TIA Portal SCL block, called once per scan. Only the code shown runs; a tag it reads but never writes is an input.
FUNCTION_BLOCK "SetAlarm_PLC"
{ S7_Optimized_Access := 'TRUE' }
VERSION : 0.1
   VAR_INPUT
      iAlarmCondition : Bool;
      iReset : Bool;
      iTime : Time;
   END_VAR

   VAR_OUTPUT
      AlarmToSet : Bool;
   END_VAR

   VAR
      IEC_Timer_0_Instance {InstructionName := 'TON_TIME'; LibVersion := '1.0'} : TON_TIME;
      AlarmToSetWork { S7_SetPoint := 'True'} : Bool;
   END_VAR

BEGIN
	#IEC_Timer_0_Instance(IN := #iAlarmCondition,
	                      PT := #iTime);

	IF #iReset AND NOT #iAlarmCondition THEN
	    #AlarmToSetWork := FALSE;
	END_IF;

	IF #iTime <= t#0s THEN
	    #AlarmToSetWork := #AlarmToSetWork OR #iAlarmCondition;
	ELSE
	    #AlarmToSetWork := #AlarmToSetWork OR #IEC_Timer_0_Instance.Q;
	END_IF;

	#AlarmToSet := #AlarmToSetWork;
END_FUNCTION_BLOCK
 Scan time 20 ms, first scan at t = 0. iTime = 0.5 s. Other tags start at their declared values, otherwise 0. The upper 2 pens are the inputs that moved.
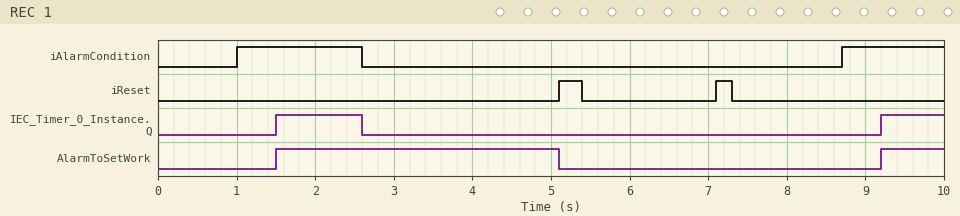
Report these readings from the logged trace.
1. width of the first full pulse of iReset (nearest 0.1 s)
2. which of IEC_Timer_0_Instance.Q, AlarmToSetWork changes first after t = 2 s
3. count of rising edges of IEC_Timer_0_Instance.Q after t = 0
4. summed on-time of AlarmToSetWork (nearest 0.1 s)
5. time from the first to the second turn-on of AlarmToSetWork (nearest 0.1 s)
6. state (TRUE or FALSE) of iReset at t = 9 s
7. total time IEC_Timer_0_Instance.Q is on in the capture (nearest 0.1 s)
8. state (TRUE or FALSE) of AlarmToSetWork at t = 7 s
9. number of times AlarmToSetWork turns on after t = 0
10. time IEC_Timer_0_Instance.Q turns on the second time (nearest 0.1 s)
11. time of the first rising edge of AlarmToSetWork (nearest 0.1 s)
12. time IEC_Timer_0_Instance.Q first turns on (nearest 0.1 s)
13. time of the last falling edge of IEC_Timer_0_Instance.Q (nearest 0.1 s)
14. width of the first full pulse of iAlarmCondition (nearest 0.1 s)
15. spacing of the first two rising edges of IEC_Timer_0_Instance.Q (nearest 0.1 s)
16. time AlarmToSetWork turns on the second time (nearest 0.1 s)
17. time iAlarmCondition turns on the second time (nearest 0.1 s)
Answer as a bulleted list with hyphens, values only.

- 0.3 s
- IEC_Timer_0_Instance.Q
- 2
- 4.4 s
- 7.7 s
- FALSE
- 1.9 s
- FALSE
- 2
- 9.2 s
- 1.5 s
- 1.5 s
- 2.6 s
- 1.6 s
- 7.7 s
- 9.2 s
- 8.7 s
